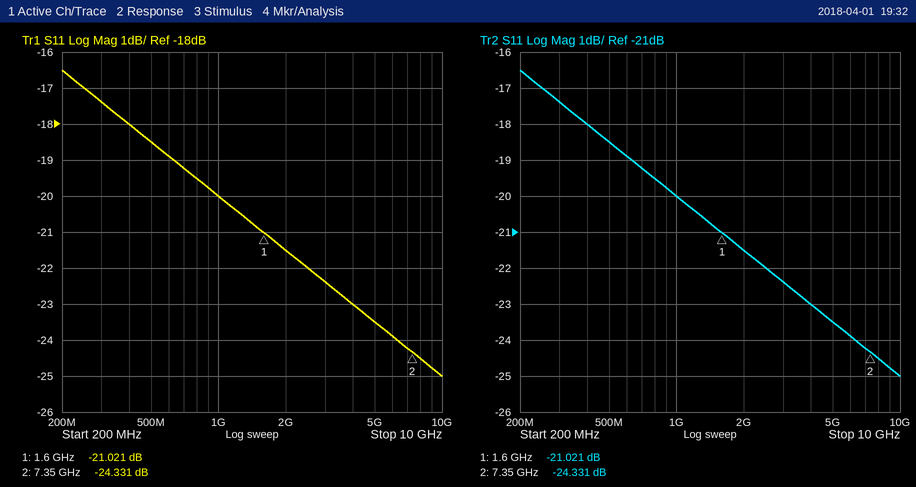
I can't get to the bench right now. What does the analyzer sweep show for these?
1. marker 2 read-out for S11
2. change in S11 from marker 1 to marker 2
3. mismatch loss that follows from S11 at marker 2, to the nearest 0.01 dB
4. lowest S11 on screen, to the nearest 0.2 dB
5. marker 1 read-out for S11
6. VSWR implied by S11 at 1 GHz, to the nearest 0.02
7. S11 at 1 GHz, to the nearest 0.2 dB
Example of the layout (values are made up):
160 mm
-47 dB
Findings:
-24.331 dB
-3.310 dB
0.02 dB
-25.0 dB
-21.021 dB
1.22
-20.0 dB
